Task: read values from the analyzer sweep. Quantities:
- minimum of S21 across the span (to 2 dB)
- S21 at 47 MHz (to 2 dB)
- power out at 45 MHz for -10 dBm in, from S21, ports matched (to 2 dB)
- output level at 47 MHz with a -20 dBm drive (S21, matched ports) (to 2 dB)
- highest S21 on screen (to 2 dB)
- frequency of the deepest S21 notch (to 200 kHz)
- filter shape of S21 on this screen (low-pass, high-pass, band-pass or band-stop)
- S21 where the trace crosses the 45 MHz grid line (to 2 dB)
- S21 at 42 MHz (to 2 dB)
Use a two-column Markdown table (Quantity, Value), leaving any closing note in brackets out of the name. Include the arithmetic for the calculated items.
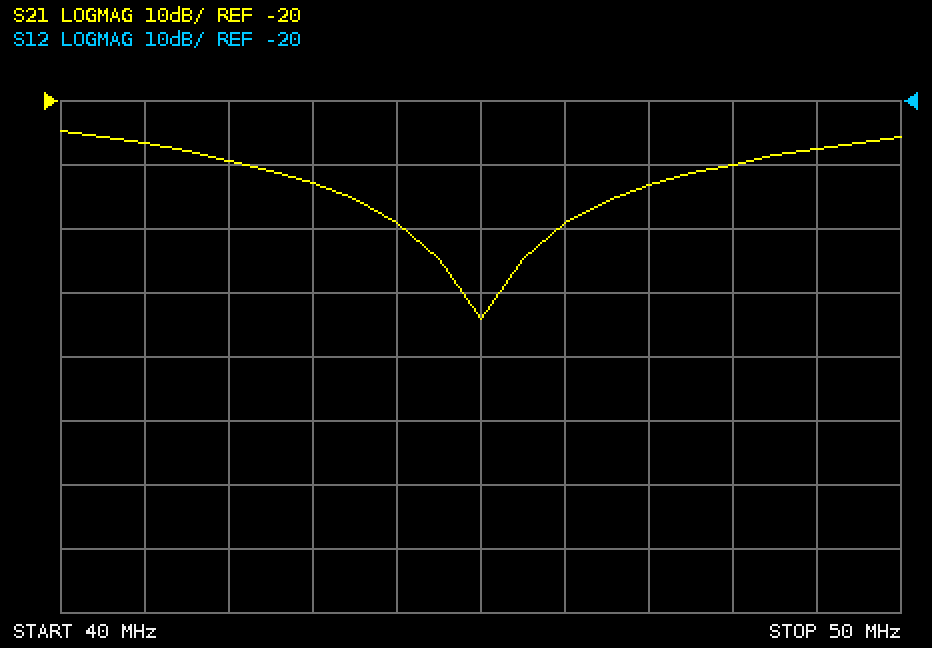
| Quantity | Value |
|---|---|
| minimum of S21 across the span | -54 dB |
| S21 at 47 MHz | -34 dB |
| power out at 45 MHz for -10 dBm in, from S21, ports matched | -10 dBm + (-54 dB) = -64 dBm |
| output level at 47 MHz with a -20 dBm drive (S21, matched ports) | -20 dBm + (-34 dB) = -54 dBm |
| highest S21 on screen | -24 dB |
| frequency of the deepest S21 notch | 45.0 MHz |
| filter shape of S21 on this screen | band-stop |
| S21 where the trace crosses the 45 MHz grid line | -54 dB |
| S21 at 42 MHz | -30 dB |
